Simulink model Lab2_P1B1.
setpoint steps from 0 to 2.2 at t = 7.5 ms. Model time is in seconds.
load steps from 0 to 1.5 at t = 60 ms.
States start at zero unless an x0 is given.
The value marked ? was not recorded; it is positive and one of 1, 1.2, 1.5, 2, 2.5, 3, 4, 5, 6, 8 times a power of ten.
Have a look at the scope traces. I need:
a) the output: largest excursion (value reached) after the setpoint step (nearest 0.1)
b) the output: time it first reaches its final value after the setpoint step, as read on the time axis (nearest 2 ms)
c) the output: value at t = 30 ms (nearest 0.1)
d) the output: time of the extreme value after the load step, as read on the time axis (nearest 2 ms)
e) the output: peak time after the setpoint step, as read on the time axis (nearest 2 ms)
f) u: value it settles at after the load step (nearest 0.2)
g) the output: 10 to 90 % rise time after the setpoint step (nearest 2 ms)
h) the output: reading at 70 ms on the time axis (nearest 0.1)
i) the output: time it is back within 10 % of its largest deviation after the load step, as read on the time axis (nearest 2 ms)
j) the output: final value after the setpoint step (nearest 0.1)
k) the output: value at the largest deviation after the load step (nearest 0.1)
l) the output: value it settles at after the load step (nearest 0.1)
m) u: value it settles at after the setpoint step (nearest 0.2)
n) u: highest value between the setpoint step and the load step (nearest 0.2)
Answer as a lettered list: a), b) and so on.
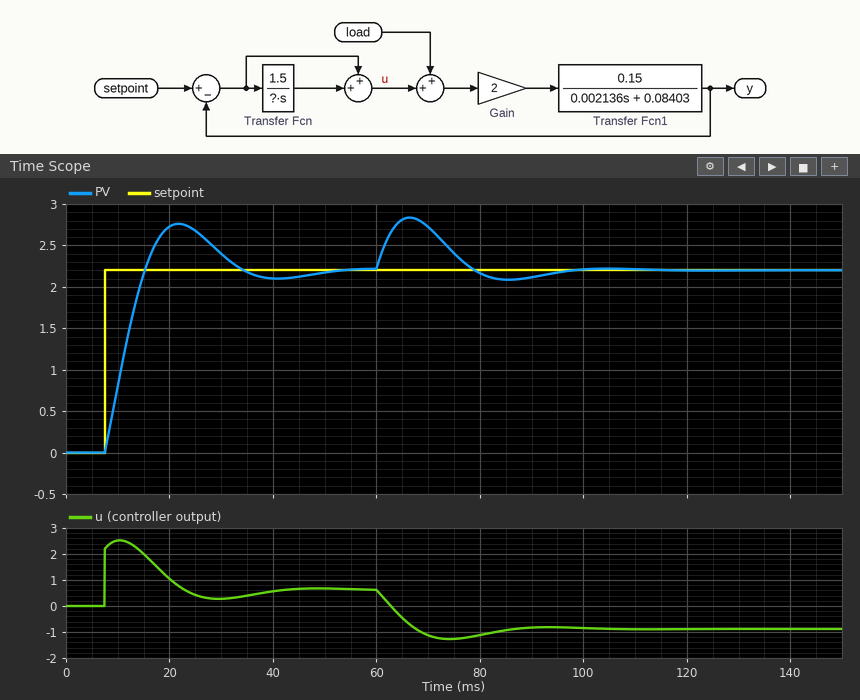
a) 2.8
b) 16 ms
c) 2.4
d) 66 ms
e) 22 ms
f) -0.8
g) 6 ms
h) 2.7
i) 92 ms
j) 2.2
k) 2.8
l) 2.2
m) 0.6
n) 2.6
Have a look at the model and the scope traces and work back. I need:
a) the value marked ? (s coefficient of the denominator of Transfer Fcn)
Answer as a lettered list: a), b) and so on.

a) 0.006
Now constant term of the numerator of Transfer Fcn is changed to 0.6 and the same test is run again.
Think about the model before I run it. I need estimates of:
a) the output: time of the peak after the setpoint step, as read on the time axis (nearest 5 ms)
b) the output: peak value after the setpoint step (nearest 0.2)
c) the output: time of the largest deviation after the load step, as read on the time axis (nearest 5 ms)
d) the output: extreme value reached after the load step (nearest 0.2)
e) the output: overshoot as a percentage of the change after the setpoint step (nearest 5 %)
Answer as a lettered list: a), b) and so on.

a) 30 ms
b) 2.4
c) 70 ms
d) 3.0
e) 10 %
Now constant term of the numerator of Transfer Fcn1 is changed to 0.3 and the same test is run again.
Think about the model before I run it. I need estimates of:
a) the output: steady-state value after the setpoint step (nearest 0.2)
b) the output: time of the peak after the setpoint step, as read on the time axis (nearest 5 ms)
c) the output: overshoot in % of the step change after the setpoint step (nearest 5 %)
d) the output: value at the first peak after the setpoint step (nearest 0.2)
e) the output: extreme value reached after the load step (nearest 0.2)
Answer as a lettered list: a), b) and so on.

a) 2.2
b) 15 ms
c) 20 %
d) 2.6
e) 3.0
